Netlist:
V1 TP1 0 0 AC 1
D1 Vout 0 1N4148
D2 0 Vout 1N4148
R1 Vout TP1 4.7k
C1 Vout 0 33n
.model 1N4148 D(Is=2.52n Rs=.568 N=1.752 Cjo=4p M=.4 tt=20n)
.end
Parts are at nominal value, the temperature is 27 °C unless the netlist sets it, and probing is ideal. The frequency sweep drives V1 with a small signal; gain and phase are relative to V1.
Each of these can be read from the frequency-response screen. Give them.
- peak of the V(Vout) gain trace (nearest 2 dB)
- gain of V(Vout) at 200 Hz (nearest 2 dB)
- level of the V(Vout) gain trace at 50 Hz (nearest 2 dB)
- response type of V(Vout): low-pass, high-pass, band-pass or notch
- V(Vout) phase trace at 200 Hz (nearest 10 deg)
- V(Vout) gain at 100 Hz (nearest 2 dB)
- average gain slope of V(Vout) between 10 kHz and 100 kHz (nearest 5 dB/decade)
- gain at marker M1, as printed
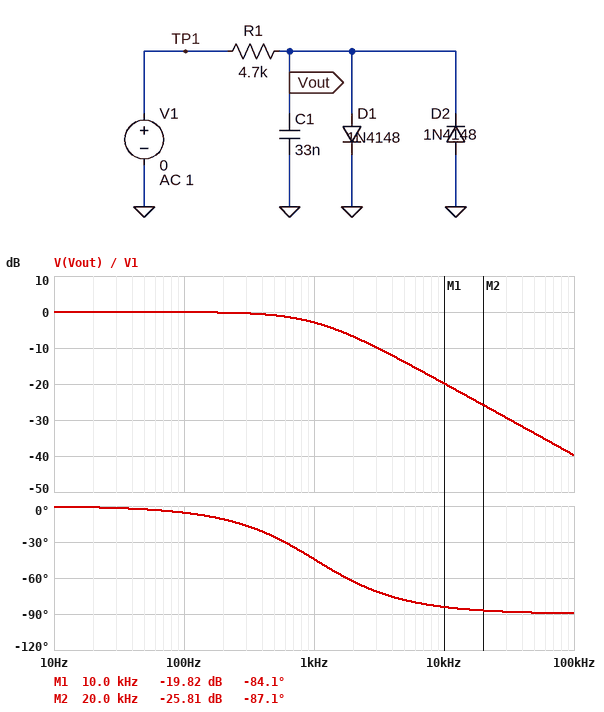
0 dB
0 dB
0 dB
low-pass
-10 deg
0 dB
-20 dB/decade
-19.82 dB
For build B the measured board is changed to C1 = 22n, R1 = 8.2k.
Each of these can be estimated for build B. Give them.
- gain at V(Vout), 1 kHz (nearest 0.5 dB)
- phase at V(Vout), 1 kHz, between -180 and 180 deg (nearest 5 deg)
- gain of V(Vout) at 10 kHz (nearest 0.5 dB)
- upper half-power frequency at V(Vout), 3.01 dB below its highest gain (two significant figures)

-3.5 dB
-50 deg
-21.0 dB
880 Hz
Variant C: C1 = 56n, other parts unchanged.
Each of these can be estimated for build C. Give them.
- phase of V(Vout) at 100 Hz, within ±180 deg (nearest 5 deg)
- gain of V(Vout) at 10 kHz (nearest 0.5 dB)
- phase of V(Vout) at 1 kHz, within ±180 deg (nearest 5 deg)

-10 deg
-24.5 dB
-60 deg
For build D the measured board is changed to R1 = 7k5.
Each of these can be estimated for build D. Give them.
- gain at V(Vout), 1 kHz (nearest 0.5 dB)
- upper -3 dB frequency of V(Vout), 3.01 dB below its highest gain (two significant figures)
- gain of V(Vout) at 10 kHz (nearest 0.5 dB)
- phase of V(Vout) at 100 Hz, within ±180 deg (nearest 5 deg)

-5.5 dB
640 Hz
-24.0 dB
-10 deg
